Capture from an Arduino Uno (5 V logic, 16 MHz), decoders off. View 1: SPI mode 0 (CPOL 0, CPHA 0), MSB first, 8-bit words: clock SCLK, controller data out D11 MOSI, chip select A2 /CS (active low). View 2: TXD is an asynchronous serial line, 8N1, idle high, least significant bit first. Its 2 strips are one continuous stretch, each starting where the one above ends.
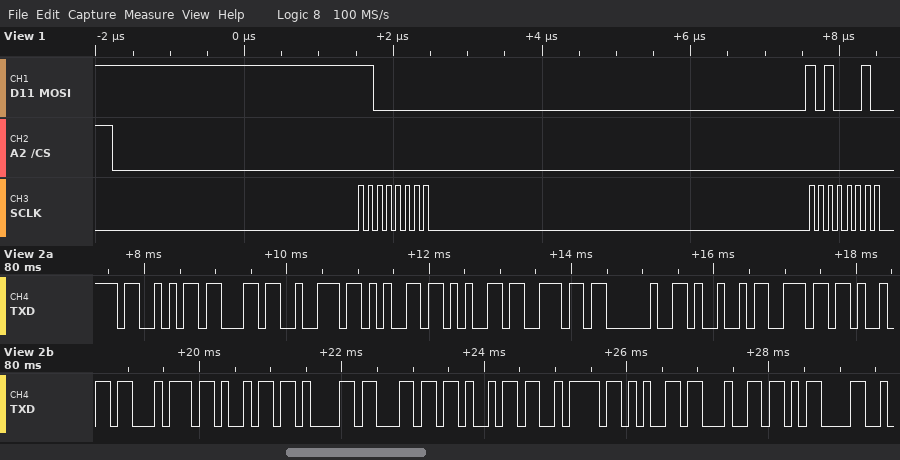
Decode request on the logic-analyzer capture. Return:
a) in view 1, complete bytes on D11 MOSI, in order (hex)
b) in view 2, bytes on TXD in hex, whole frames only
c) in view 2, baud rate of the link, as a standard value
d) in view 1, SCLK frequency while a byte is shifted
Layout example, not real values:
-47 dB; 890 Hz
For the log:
0xC0 0xA2; 53 63 72 65 65 6E 20 49 6E 69 74 69 61 6C 69 7A 65 64 0D; 9600 baud; 8 MHz
